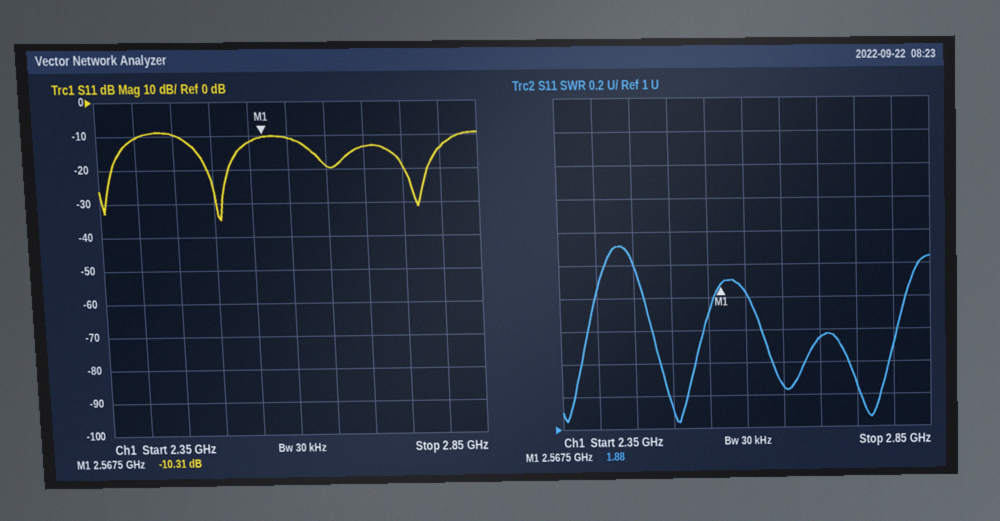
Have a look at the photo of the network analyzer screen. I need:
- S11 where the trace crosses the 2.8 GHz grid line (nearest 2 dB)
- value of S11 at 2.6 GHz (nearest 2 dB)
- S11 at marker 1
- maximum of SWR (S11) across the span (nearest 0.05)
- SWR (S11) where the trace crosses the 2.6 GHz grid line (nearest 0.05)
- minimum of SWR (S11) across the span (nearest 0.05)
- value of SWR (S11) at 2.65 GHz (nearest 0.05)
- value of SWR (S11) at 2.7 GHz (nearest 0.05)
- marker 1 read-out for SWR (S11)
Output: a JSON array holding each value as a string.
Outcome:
["-14 dB", "-10 dB", "-10.31 dB", "2.10", "1.85", "1.05", "1.25", "1.55", "1.88"]
